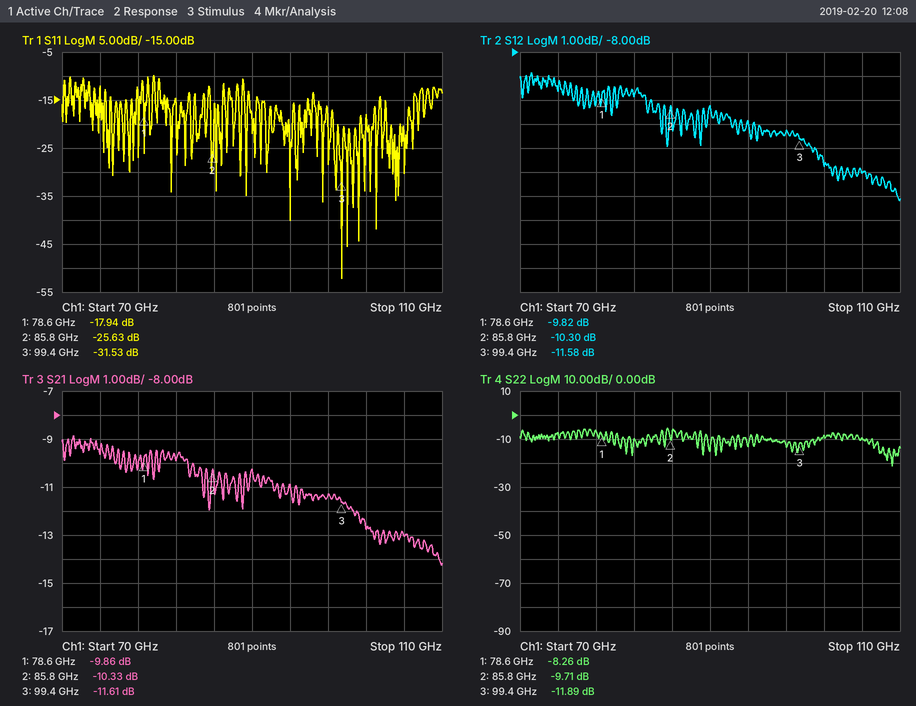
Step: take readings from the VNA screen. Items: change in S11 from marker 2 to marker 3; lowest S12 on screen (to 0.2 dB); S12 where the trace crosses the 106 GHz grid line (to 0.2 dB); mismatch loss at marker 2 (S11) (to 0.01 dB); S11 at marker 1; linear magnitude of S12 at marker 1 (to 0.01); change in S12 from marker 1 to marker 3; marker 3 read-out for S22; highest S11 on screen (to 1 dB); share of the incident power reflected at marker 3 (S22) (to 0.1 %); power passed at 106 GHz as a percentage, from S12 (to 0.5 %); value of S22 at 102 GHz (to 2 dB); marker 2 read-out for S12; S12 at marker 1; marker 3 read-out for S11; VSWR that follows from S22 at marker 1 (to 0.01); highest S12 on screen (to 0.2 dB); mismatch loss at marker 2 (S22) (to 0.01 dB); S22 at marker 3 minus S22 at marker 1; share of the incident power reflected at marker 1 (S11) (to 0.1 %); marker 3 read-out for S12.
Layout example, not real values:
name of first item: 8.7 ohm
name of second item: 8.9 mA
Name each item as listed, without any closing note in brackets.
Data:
change in S11 from marker 2 to marker 3: -5.90 dB
lowest S12 on screen: -14.2 dB
S12 where the trace crosses the 106 GHz grid line: -13.0 dB
mismatch loss at marker 2 (S11): 0.01 dB
S11 at marker 1: -17.94 dB
linear magnitude of S12 at marker 1: 0.32
change in S12 from marker 1 to marker 3: -1.76 dB
marker 3 read-out for S22: -11.89 dB
highest S11 on screen: -10 dB
share of the incident power reflected at marker 3 (S22): 6.5 %
power passed at 106 GHz as a percentage, from S12: 5.0 %
value of S22 at 102 GHz: -8 dB
marker 2 read-out for S12: -10.30 dB
S12 at marker 1: -9.82 dB
marker 3 read-out for S11: -31.53 dB
VSWR that follows from S22 at marker 1: 2.26
highest S12 on screen: -8.8 dB
mismatch loss at marker 2 (S22): 0.49 dB
S22 at marker 3 minus S22 at marker 1: -3.63 dB
share of the incident power reflected at marker 1 (S11): 1.6 %
marker 3 read-out for S12: -11.58 dB
